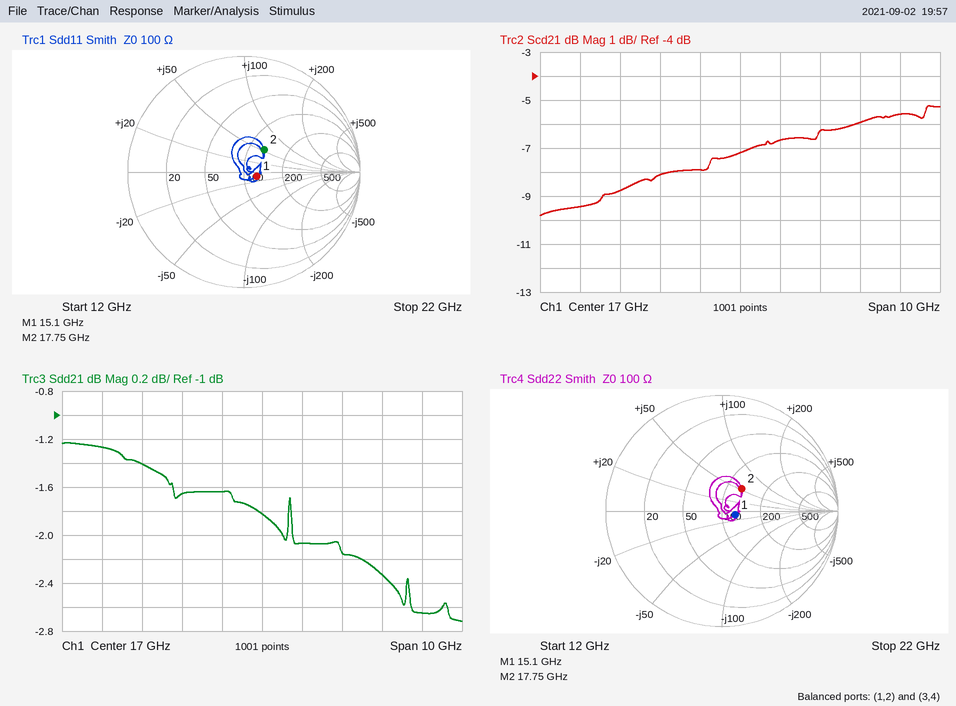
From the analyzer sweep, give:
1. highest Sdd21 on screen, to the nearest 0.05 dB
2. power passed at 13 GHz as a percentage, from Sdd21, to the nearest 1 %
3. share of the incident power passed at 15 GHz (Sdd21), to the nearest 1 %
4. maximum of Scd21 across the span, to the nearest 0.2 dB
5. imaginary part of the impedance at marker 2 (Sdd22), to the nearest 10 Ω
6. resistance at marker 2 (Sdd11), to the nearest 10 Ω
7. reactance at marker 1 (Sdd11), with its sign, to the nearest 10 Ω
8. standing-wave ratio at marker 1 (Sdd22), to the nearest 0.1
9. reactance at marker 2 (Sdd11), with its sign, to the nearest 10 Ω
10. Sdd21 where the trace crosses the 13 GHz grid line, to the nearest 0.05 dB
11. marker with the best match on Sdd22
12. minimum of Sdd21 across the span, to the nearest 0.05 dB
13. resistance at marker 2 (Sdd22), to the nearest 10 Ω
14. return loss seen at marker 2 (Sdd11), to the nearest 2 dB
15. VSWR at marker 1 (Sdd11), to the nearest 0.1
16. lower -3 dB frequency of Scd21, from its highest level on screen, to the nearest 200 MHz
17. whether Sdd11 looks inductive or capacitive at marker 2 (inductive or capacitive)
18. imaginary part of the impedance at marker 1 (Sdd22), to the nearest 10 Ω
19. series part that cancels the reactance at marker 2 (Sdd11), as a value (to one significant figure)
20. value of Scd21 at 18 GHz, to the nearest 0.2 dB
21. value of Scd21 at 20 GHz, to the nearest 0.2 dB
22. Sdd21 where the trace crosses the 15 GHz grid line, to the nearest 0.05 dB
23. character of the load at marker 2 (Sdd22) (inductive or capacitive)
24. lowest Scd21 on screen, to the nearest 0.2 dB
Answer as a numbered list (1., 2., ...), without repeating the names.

1. -1.25 dB
2. 75 %
3. 68 %
4. -5.2 dB
5. +50 Ω
6. 130 Ω
7. -10 Ω
8. 1.3
9. +50 Ω
10. -1.25 dB
11. marker 1
12. -2.70 dB
13. 130 Ω
14. 12 dB
15. 1.3
16. 14.8 GHz
17. inductive
18. -10 Ω
19. 200 fF
20. -6.6 dB
21. -6.0 dB
22. -1.65 dB
23. inductive
24. -9.8 dB
